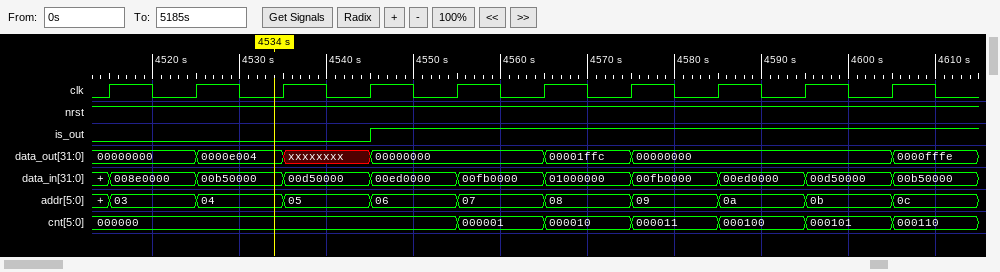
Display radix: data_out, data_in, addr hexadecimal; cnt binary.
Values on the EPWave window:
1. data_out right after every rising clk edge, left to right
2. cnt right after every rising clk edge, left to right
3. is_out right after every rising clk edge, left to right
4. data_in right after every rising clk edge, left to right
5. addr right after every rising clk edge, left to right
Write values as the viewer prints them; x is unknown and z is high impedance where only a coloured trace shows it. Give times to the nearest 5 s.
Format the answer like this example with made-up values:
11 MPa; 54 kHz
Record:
00000000, 0000e004, xxxxxxxx, 00000000, 00000000, 00001ffc, 00000000, 00000000, 00000000, 0000fffe; 000000, 000000, 000000, 000000, 000001, 000010, 000011, 000100, 000101, 000110; 0 0 0 1 1 1 1 1 1 1; 008e0000, 00b50000, 00d50000, 00ed0000, 00fb0000, 01000000, 00fb0000, 00ed0000, 00d50000, 00b50000; 03, 04, 05, 06, 07, 08, 09, 0a, 0b, 0c
